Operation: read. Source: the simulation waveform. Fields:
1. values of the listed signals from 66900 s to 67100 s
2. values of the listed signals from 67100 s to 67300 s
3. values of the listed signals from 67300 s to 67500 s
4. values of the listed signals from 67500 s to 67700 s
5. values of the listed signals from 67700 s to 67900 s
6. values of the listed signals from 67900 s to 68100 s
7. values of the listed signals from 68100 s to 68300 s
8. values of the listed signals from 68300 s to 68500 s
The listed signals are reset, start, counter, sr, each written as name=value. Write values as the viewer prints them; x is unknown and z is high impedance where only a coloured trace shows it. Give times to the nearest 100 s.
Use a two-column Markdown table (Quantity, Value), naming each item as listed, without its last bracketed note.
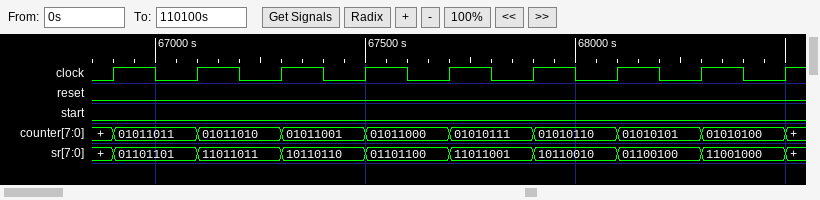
| Quantity | Value |
|---|---|
| values of the listed signals from 66900 s to 67100 s | reset=0, start=0, counter=01011011, sr=01101101 |
| values of the listed signals from 67100 s to 67300 s | reset=0, start=0, counter=01011010, sr=11011011 |
| values of the listed signals from 67300 s to 67500 s | reset=0, start=0, counter=01011001, sr=10110110 |
| values of the listed signals from 67500 s to 67700 s | reset=0, start=0, counter=01011000, sr=01101100 |
| values of the listed signals from 67700 s to 67900 s | reset=0, start=0, counter=01010111, sr=11011001 |
| values of the listed signals from 67900 s to 68100 s | reset=0, start=0, counter=01010110, sr=10110010 |
| values of the listed signals from 68100 s to 68300 s | reset=0, start=0, counter=01010101, sr=01100100 |
| values of the listed signals from 68300 s to 68500 s | reset=0, start=0, counter=01010100, sr=11001000 |
